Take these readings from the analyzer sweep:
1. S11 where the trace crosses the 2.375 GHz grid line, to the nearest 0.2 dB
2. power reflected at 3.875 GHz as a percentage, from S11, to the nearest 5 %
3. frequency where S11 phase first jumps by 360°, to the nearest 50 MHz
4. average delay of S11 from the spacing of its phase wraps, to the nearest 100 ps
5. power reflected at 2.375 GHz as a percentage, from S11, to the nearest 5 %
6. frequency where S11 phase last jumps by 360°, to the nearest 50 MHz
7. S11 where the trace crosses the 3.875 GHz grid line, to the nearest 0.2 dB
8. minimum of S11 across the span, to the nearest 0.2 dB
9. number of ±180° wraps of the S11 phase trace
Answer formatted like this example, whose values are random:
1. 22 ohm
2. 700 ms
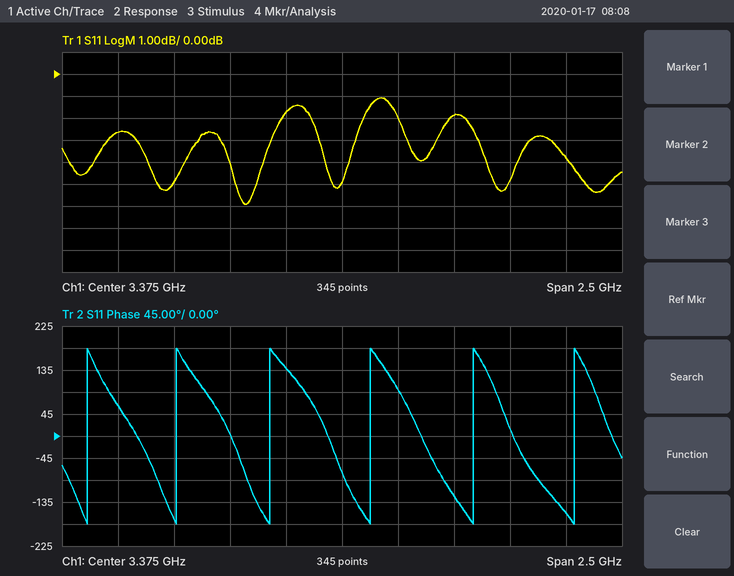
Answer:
1. -2.6 dB
2. 65 %
3. 2.25 GHz
4. 2.3 ns
5. 55 %
6. 4.40 GHz
7. -1.8 dB
8. -6.0 dB
9. 6
